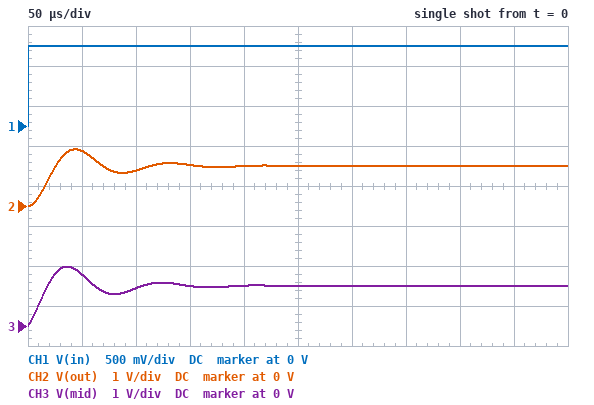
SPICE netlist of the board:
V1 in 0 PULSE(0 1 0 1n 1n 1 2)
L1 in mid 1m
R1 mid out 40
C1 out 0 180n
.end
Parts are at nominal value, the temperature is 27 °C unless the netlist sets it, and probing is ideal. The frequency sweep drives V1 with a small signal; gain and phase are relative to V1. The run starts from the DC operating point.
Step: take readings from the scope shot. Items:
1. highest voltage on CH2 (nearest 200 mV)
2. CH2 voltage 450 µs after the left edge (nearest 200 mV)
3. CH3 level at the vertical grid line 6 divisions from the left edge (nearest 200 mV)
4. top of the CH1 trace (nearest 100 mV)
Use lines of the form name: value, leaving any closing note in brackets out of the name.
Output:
highest voltage on CH2: 1.4 V
CH2 voltage 450 µs after the left edge: 1.0 V
CH3 level at the vertical grid line 6 divisions from the left edge: 1.0 V
top of the CH1 trace: 1.0 V
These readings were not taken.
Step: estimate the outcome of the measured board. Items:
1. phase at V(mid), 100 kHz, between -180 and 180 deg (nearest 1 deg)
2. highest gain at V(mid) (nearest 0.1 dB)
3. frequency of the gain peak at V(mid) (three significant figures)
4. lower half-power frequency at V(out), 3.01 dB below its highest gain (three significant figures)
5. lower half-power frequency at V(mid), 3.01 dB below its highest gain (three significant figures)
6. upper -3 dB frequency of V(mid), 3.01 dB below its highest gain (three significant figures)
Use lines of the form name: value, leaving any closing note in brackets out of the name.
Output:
phase at V(mid), 100 kHz, between -180 and 180 deg: -99 deg
highest gain at V(mid): 6.7 dB
frequency of the gain peak at V(mid): 11.2 kHz
lower half-power frequency at V(out), 3.01 dB below its highest gain: 6.91 kHz
lower half-power frequency at V(mid), 3.01 dB below its highest gain: 7.49 kHz
upper -3 dB frequency of V(mid), 3.01 dB below its highest gain: 14.2 kHz
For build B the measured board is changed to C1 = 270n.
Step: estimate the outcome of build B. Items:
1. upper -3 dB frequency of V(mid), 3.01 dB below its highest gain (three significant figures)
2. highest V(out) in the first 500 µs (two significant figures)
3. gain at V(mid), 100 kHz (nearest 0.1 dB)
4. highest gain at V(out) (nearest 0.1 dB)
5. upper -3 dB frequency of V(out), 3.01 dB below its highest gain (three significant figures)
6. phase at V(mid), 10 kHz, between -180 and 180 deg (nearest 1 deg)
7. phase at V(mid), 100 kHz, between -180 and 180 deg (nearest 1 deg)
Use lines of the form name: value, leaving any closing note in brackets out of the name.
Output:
upper -3 dB frequency of V(mid), 3.01 dB below its highest gain: 12.0 kHz
highest V(out) in the first 500 µs: 1.3 V
gain at V(mid), 100 kHz: -23.8 dB
highest gain at V(out): 4.1 dB
upper -3 dB frequency of V(out), 3.01 dB below its highest gain: 11.5 kHz
phase at V(mid), 10 kHz, between -180 and 180 deg: -61 deg
phase at V(mid), 100 kHz, between -180 and 180 deg: -95 deg
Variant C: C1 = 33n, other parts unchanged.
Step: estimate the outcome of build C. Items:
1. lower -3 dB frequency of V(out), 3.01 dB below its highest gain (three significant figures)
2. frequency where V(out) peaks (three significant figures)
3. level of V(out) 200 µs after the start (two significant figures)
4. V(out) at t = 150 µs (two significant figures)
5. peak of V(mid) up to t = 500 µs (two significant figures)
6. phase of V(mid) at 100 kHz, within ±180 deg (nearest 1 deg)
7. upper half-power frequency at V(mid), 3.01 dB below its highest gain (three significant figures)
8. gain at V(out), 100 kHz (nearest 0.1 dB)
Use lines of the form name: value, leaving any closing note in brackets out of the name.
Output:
lower -3 dB frequency of V(out), 3.01 dB below its highest gain: 23.9 kHz
frequency where V(out) peaks: 27.3 kHz
level of V(out) 200 µs after the start: 1.0 V
V(out) at t = 150 µs: 960 mV
peak of V(mid) up to t = 500 µs: 1.7 V
phase of V(mid) at 100 kHz, within ±180 deg: -136 deg
upper half-power frequency at V(mid), 3.01 dB below its highest gain: 30.4 kHz
gain at V(out), 100 kHz: -21.6 dB
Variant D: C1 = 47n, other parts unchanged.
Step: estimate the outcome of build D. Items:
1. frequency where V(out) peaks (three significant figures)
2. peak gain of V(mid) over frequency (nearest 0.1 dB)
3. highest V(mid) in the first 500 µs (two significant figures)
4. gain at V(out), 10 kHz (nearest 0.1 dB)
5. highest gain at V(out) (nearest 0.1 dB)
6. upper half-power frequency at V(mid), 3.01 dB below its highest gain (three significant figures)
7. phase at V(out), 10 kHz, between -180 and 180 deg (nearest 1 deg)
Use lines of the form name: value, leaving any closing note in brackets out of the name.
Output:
frequency where V(out) peaks: 22.8 kHz
peak gain of V(mid) over frequency: 11.6 dB
highest V(mid) in the first 500 µs: 1.7 V
gain at V(out), 10 kHz: 1.7 dB
highest gain at V(out): 11.3 dB
upper half-power frequency at V(mid), 3.01 dB below its highest gain: 25.8 kHz
phase at V(out), 10 kHz, between -180 and 180 deg: -8 deg
